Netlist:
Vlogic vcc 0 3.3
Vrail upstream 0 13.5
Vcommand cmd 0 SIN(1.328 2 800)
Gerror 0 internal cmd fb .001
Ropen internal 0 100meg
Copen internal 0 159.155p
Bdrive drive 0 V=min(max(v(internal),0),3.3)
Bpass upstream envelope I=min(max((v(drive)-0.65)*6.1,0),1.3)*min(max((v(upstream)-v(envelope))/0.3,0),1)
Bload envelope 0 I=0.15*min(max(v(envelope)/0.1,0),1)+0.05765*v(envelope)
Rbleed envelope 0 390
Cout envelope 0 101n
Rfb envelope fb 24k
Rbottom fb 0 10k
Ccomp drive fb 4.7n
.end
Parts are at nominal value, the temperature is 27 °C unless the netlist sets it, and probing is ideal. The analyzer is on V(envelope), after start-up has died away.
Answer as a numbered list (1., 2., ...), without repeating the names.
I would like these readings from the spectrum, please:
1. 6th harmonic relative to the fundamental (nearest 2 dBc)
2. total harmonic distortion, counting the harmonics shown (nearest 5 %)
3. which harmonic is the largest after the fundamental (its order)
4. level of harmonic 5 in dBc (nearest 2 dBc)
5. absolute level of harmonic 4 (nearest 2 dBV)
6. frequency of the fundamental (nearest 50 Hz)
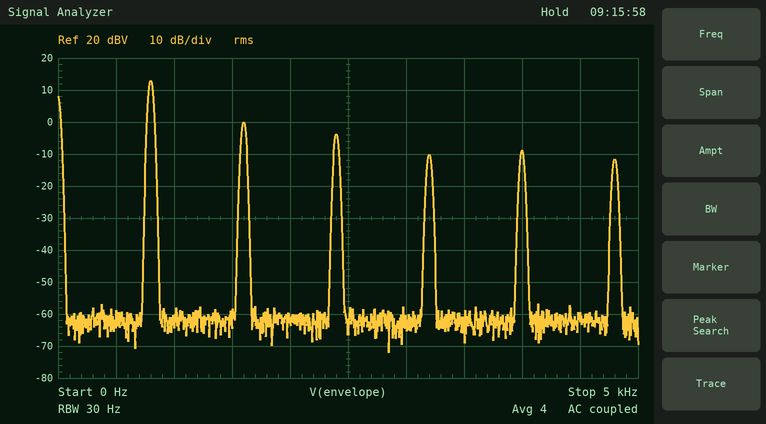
1. -24 dBc
2. 30 %
3. 2
4. -22 dBc
5. -10 dBV
6. 800 Hz
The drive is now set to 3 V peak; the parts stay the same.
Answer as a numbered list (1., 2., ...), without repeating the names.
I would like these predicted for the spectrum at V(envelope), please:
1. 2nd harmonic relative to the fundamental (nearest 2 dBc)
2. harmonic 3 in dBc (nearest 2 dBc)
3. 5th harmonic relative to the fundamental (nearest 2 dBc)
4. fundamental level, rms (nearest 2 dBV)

1. -6 dBc
2. -28 dBc
3. -16 dBc
4. 14 dBV
